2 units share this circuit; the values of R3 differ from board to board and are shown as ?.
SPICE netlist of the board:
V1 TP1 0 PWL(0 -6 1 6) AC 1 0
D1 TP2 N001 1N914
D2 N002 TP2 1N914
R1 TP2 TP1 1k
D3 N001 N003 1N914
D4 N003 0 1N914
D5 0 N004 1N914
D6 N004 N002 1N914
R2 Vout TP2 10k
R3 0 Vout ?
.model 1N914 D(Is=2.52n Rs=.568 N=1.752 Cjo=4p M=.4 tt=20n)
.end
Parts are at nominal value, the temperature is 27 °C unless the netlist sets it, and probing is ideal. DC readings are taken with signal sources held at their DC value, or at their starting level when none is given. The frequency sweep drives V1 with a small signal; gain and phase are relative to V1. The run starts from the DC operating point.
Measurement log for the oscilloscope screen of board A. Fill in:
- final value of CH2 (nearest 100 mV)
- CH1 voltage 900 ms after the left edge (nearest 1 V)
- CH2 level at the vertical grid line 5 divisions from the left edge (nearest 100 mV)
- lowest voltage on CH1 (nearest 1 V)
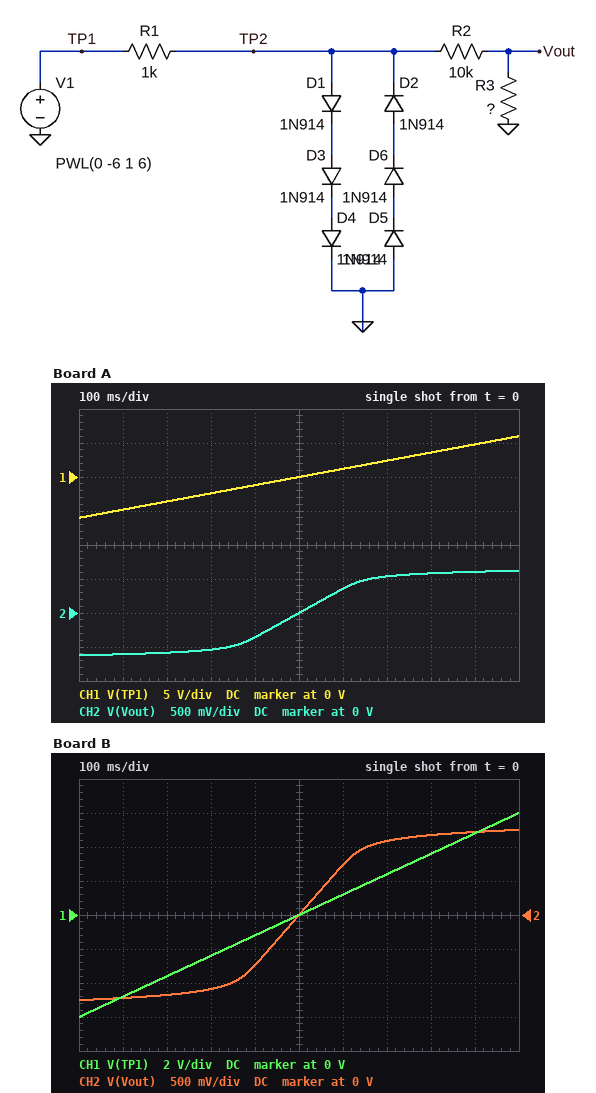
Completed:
600 mV
5 V
0 V
-6 V
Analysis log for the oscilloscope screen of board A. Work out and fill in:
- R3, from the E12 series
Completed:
4.7 kΩ
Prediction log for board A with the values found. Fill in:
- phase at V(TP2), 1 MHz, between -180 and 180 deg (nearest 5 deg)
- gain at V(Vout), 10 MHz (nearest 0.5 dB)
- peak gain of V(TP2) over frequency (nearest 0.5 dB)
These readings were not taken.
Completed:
-5 deg
-43.0 dB
-29.0 dB
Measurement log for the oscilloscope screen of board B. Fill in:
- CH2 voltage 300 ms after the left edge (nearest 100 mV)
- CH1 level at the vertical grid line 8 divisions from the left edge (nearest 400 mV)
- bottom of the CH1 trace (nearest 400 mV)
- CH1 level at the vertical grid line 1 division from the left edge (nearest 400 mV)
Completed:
-1.1 V
3.6 V
-6.0 V
-4.8 V
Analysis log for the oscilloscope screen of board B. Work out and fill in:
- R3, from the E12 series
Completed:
18 kΩ
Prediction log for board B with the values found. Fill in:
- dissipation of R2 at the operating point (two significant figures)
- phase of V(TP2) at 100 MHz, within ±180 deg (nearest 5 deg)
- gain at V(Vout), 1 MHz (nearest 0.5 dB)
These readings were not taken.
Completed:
48 µW
-55 deg
-33.0 dB
